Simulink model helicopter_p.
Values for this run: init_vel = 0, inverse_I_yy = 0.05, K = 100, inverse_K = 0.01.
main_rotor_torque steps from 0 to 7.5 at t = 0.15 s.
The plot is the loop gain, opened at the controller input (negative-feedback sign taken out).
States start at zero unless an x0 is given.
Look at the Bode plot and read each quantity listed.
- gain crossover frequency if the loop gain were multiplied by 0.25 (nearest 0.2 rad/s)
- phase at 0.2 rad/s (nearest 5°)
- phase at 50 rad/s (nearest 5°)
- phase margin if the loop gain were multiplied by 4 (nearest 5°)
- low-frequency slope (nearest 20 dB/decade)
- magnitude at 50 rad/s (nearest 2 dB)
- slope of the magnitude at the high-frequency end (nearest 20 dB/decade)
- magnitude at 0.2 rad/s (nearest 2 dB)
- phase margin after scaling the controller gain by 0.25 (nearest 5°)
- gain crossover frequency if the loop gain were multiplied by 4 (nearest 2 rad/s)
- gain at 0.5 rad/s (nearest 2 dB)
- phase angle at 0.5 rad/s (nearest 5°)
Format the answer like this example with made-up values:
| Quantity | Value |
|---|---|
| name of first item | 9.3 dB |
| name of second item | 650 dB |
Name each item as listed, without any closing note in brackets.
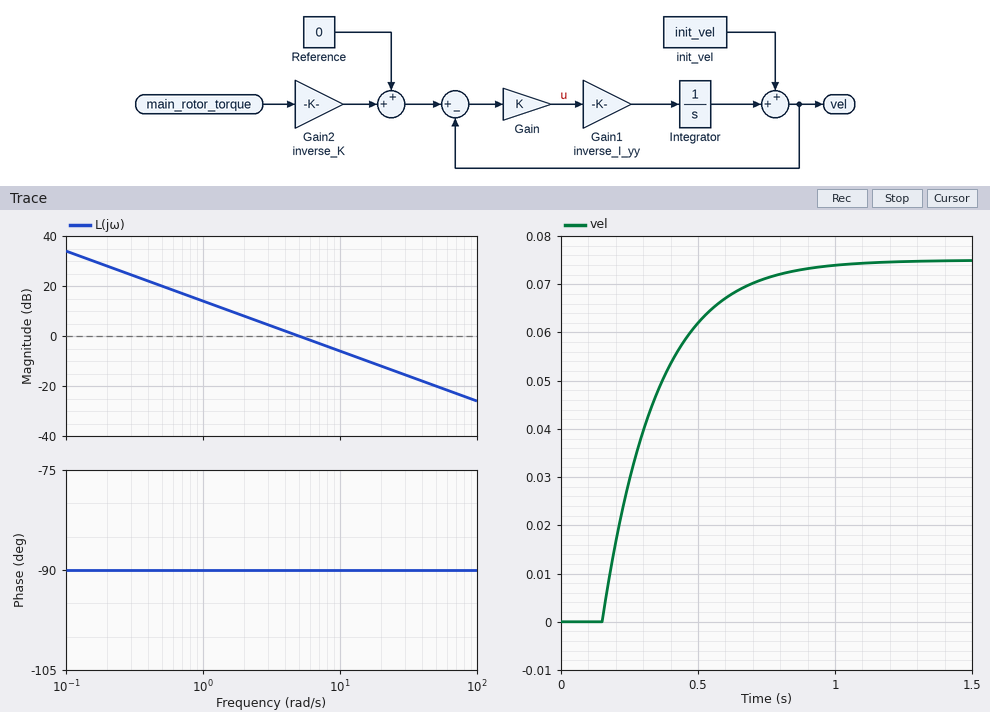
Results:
| Quantity | Value |
|---|---|
| gain crossover frequency if the loop gain were multiplied by 0.25 | 1.2 rad/s |
| phase at 0.2 rad/s | -90° |
| phase at 50 rad/s | -90° |
| phase margin if the loop gain were multiplied by 4 | 90° |
| low-frequency slope | -20 dB/decade |
| magnitude at 50 rad/s | -20 dB |
| slope of the magnitude at the high-frequency end | -20 dB/decade |
| magnitude at 0.2 rad/s | 28 dB |
| phase margin after scaling the controller gain by 0.25 | 90° |
| gain crossover frequency if the loop gain were multiplied by 4 | 20 rad/s |
| gain at 0.5 rad/s | 20 dB |
| phase angle at 0.5 rad/s | -90° |
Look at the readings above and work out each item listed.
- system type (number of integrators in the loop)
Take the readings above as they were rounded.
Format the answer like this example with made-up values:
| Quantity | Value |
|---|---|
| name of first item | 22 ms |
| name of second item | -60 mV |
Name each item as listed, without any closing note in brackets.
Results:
| Quantity | Value |
|---|---|
| system type | 1 |
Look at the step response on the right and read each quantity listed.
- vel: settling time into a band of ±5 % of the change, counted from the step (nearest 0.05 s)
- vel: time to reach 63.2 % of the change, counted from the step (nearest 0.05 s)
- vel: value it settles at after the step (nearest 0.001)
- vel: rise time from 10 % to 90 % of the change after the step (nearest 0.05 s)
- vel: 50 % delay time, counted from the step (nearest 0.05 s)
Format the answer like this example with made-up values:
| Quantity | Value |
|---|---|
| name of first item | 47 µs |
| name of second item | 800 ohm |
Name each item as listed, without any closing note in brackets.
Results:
| Quantity | Value |
|---|---|
| vel: settling time into a band of ±5 % of the change, counted from the step | 0.60 s |
| vel: time to reach 63.2 % of the change, counted from the step | 0.20 s |
| vel: value it settles at after the step | 0.075 |
| vel: rise time from 10 % to 90 % of the change after the step | 0.45 s |
| vel: 50 % delay time, counted from the step | 0.15 s |
